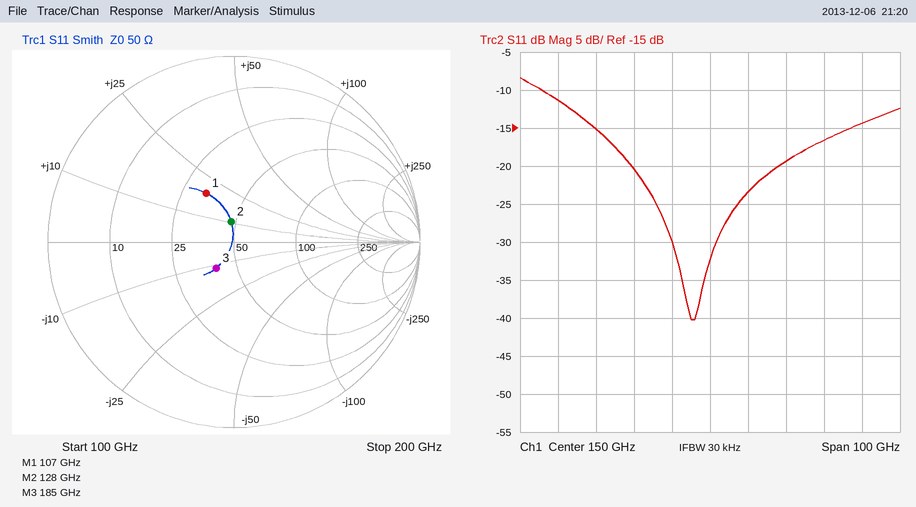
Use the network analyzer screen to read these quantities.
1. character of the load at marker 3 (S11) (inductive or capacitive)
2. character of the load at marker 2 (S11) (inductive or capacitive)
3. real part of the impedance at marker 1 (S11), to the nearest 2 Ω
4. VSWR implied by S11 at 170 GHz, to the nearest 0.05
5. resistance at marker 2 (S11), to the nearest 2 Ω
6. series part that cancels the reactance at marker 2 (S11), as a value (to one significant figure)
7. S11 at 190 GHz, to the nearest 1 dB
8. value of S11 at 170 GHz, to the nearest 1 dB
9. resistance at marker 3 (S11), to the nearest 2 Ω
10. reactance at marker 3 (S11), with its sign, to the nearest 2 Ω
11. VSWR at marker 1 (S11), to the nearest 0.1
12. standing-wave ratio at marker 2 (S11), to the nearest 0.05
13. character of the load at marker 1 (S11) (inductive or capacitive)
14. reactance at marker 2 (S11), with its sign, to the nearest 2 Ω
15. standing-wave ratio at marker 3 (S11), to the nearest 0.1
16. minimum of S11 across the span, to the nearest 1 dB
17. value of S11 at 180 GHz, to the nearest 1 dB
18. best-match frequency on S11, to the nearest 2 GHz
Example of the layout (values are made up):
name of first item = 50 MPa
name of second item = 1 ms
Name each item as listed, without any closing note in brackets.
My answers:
character of the load at marker 3 (S11) = capacitive
character of the load at marker 2 (S11) = inductive
real part of the impedance at marker 1 (S11), to the nearest 2 Ω = 32 Ω
VSWR implied by S11 at 170 GHz, to the nearest 0.05 = 1.25
resistance at marker 2 (S11), to the nearest 2 Ω = 48 Ω
series part that cancels the reactance at marker 2 (S11), as a value = 100 fF
S11 at 190 GHz, to the nearest 1 dB = -14 dB
value of S11 at 170 GHz, to the nearest 1 dB = -19 dB
resistance at marker 3 (S11), to the nearest 2 Ω = 40 Ω
reactance at marker 3 (S11), with its sign, to the nearest 2 Ω = -12 Ω
VSWR at marker 1 (S11), to the nearest 0.1 = 1.9
standing-wave ratio at marker 2 (S11), to the nearest 0.05 = 1.25
character of the load at marker 1 (S11) = inductive
reactance at marker 2 (S11), with its sign, to the nearest 2 Ω = +10 Ω
standing-wave ratio at marker 3 (S11), to the nearest 0.1 = 1.4
minimum of S11 across the span, to the nearest 1 dB = -40 dB
value of S11 at 180 GHz, to the nearest 1 dB = -17 dB
best-match frequency on S11, to the nearest 2 GHz = 146 GHz
